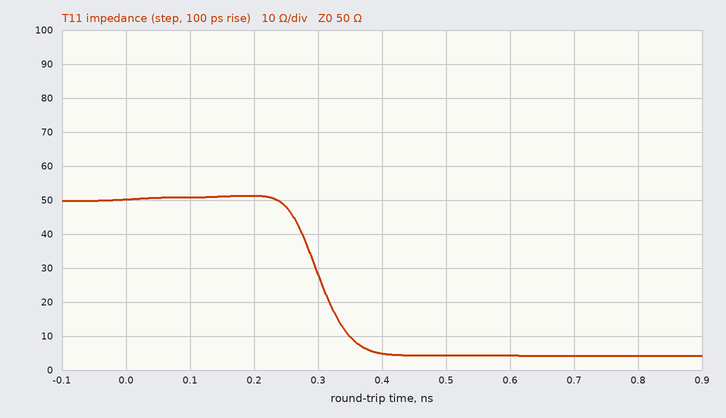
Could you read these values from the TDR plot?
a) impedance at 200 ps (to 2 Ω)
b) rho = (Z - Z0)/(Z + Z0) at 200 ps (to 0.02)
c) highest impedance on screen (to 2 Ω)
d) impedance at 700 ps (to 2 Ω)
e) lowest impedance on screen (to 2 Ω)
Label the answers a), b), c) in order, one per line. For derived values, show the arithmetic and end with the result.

a) 52 Ω
b) (52 − 50)/(52 + 50) ≈ +0.02
c) 52 Ω
d) 4 Ω
e) 4 Ω
